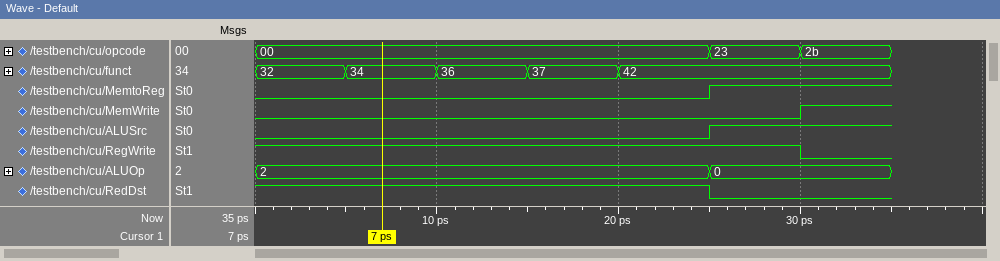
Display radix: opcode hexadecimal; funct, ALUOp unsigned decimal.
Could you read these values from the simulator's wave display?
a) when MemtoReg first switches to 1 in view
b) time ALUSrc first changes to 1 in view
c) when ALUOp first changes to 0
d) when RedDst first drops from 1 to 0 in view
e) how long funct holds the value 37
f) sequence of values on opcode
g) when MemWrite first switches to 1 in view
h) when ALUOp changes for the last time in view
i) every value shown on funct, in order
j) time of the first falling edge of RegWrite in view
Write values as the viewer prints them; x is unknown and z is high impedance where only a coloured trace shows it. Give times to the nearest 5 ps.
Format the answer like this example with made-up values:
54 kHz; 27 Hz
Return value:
25 ps; 25 ps; 25 ps; 25 ps; 5 ps; 00, 23, 2b; 30 ps; 25 ps; 32, 34, 36, 37, 42; 30 ps
